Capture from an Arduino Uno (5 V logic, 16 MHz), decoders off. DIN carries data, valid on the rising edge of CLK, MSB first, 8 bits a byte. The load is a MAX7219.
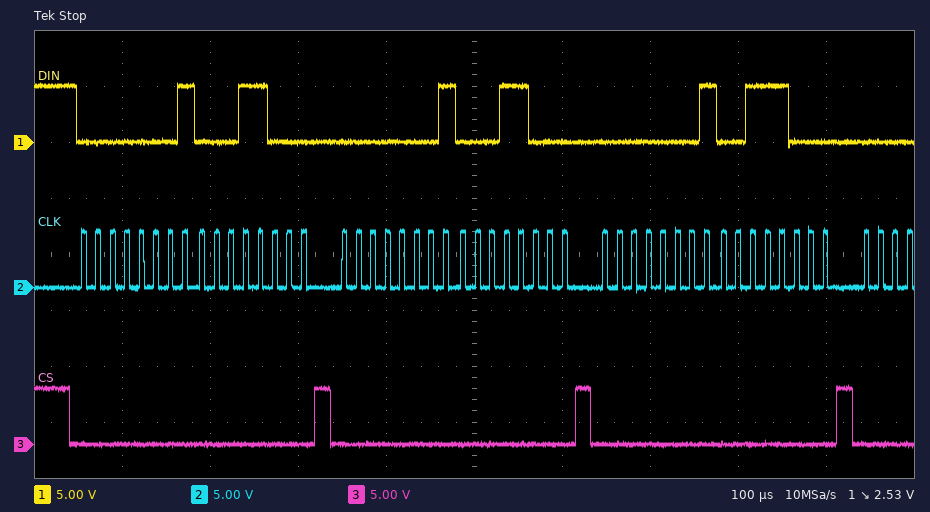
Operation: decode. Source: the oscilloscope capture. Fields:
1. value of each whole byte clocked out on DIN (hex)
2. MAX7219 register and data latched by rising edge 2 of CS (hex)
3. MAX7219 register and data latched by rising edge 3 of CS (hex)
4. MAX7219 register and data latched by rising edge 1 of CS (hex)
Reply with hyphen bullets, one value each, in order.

- 01 18 01 18 01 38
- register 0x1, data 0x18
- register 0x1, data 0x38
- register 0x1, data 0x18
